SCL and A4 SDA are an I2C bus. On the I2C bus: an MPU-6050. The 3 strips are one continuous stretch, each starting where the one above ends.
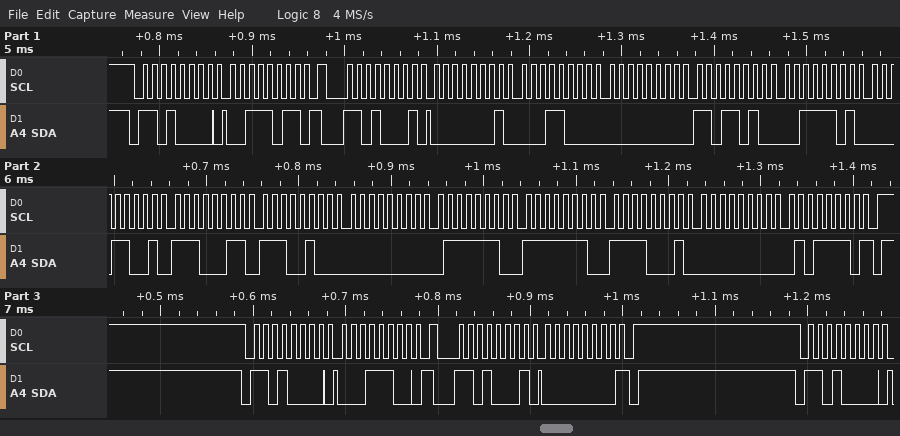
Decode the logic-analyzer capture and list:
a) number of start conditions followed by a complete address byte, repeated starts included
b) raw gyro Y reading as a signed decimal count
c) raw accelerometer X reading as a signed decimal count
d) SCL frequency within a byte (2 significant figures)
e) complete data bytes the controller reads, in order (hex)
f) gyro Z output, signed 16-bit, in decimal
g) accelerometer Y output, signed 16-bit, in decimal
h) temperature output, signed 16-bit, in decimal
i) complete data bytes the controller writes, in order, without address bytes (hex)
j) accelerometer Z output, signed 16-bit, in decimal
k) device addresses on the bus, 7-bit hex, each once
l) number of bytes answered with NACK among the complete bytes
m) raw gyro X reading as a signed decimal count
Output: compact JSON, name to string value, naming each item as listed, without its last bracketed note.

{"number of start conditions followed by a complete address byte, repeated starts included": "5", "raw gyro Y reading as a signed decimal count": "-271", "raw accelerometer X reading as a signed decimal count": "280", "SCL frequency within a byte": "100 kHz", "complete data bytes the controller reads, in order": "01 18 00 DA 3D 19 E3 E4 00 7E FE F1 00 5E 00", "gyro Z output, signed 16-bit, in decimal": "94", "accelerometer Y output, signed 16-bit, in decimal": "218", "temperature output, signed 16-bit, in decimal": "-7196", "complete data bytes the controller writes, in order, without address bytes": "3B 1C", "accelerometer Z output, signed 16-bit, in decimal": "15641", "device addresses on the bus, 7-bit hex, each once": "0x68", "number of bytes answered with NACK among the complete bytes": "2", "raw gyro X reading as a signed decimal count": "126"}
